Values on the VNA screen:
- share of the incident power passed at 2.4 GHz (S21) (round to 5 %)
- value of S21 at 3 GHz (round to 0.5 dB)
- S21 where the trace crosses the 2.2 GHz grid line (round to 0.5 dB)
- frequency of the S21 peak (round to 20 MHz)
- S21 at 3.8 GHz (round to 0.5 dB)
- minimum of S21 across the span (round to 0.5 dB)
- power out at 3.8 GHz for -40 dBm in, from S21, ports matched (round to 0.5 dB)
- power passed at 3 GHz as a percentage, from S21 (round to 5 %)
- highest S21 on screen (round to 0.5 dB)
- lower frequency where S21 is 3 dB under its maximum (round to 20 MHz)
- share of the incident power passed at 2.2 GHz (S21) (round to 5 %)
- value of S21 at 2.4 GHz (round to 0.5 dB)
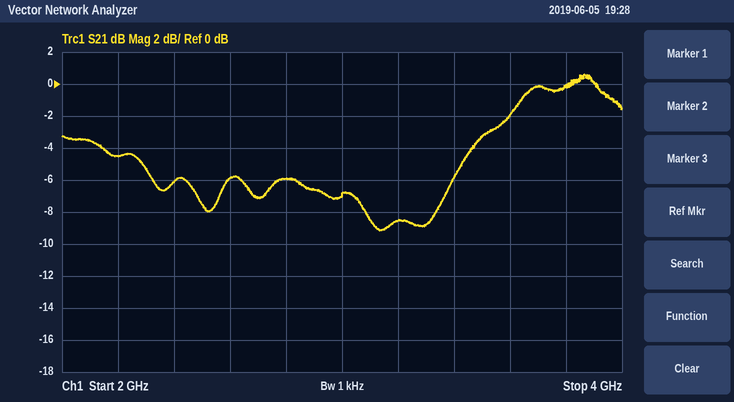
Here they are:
25 %
-7.0 dB
-4.5 dB
3.86 GHz
0.0 dB
-9.0 dB
-40.0 dBm
20 %
0.5 dB
3.58 GHz
35 %
-6.0 dB
